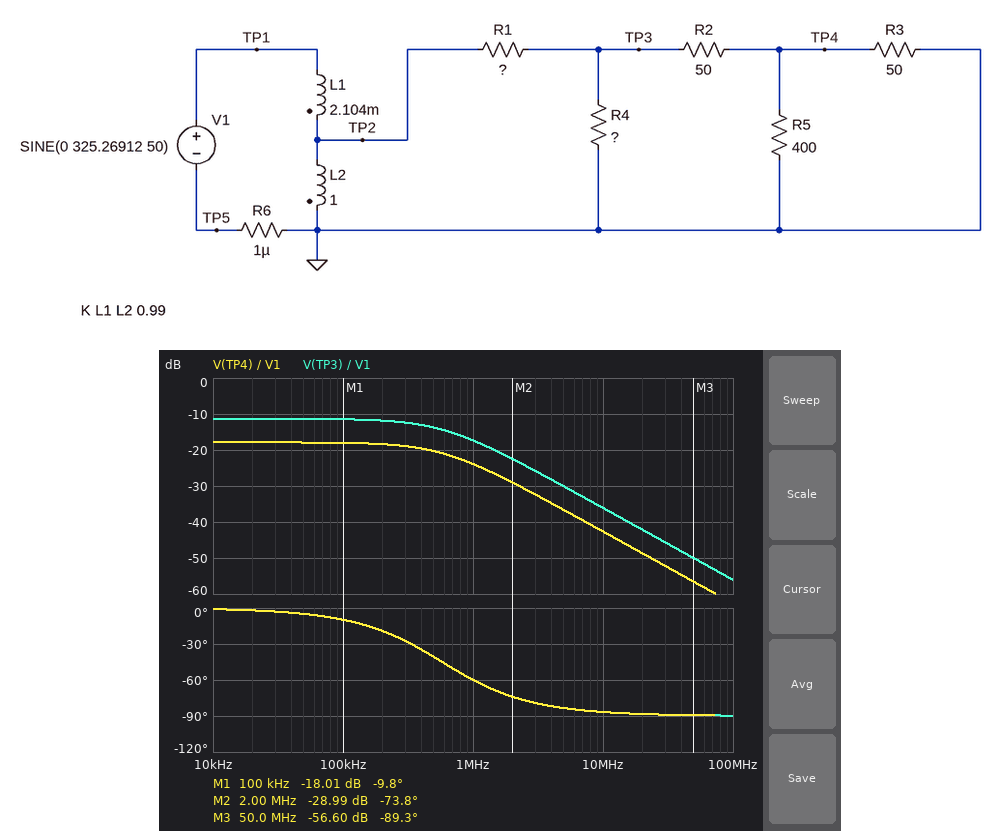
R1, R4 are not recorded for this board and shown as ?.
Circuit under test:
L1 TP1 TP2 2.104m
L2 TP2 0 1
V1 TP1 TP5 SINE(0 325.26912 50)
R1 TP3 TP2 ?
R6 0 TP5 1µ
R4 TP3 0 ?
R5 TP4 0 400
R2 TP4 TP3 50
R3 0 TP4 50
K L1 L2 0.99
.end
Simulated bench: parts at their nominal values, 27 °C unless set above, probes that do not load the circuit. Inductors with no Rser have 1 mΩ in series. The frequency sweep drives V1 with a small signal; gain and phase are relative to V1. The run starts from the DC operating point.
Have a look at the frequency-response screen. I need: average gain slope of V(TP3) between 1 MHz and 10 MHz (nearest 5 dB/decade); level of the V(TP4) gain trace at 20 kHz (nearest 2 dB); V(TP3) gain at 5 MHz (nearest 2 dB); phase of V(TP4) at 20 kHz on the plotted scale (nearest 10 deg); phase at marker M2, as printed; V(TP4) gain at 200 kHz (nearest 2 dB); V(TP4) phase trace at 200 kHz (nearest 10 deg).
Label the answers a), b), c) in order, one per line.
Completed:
a) -20 dB/decade
b) -18 dB
c) -30 dB
d) 0 deg
e) -73.8 deg
f) -18 dB
g) -20 deg
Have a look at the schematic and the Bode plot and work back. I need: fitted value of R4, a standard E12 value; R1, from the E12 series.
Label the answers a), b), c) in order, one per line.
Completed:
a) 68 Ω
b) 100 Ω
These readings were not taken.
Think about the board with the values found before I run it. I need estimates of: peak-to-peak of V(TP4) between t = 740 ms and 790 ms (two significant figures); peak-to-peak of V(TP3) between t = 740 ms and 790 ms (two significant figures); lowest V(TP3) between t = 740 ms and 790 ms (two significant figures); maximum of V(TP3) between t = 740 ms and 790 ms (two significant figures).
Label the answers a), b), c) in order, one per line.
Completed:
a) 83 V
b) 180 V
c) -88 V
d) 88 V
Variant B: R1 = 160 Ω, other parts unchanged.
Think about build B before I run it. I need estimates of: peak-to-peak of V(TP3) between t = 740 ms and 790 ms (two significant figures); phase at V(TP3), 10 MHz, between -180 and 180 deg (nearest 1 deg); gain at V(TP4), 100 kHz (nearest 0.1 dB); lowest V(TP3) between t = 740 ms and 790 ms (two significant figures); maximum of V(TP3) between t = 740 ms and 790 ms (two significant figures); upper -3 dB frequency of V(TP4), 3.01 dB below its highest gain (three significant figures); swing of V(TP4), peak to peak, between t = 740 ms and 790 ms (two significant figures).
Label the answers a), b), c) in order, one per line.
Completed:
a) 120 V
b) -85 deg
c) -21.1 dB
d) -62 V
e) 62 V
f) 829 kHz
g) 58 V
